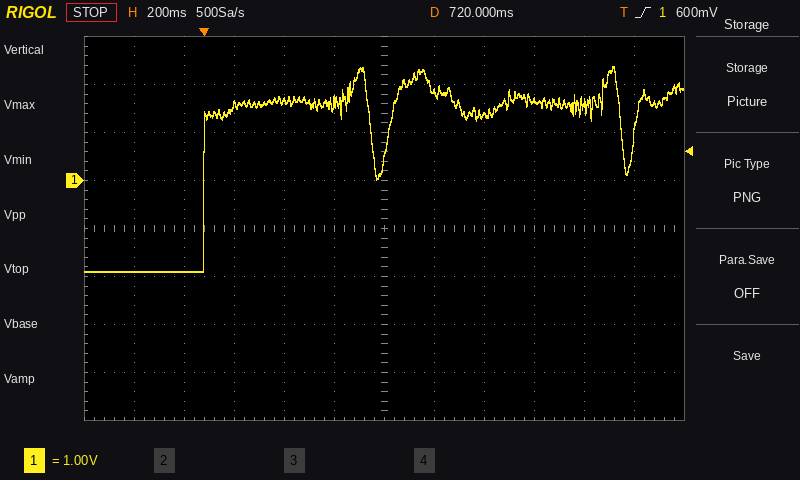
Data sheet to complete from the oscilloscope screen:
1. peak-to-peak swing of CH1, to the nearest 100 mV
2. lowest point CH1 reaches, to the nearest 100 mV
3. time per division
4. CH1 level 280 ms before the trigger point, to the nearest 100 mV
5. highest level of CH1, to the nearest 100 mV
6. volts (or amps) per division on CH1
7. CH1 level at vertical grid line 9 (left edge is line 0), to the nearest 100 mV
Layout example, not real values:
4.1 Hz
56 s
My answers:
4.3 V
-1.9 V
200 ms
-1.9 V
2.4 V
1 V
1.7 V
